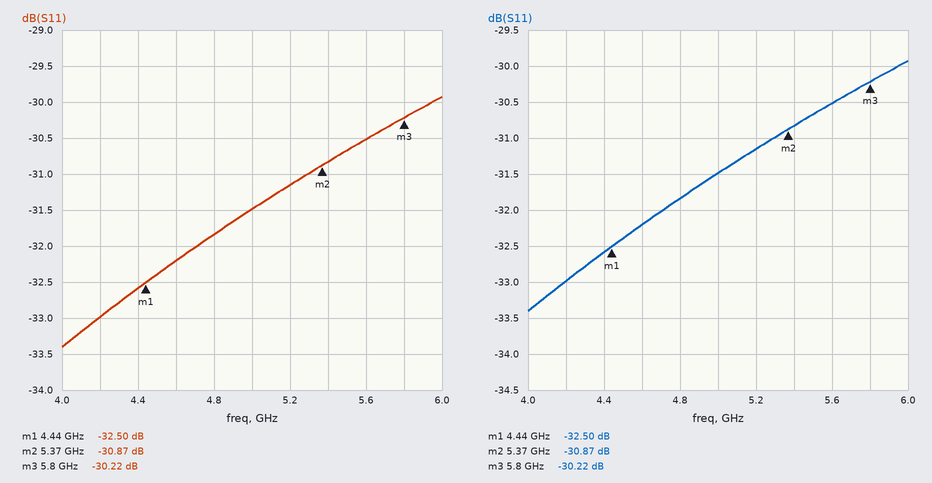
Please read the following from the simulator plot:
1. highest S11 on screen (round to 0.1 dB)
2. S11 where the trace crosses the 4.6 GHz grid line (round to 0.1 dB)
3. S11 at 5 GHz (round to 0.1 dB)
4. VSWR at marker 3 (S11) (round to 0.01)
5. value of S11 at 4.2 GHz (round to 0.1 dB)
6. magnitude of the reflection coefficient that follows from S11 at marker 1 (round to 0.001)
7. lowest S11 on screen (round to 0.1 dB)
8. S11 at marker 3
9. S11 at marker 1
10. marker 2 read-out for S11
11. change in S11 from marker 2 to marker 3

-29.9 dB
-32.2 dB
-31.5 dB
1.06
-33.0 dB
0.024
-33.4 dB
-30.22 dB
-32.50 dB
-30.87 dB
0.65 dB
